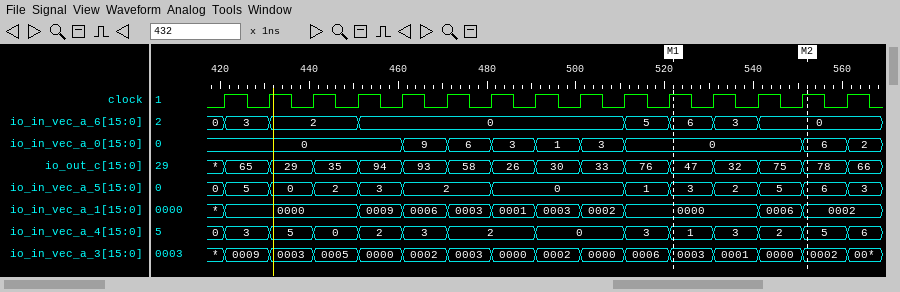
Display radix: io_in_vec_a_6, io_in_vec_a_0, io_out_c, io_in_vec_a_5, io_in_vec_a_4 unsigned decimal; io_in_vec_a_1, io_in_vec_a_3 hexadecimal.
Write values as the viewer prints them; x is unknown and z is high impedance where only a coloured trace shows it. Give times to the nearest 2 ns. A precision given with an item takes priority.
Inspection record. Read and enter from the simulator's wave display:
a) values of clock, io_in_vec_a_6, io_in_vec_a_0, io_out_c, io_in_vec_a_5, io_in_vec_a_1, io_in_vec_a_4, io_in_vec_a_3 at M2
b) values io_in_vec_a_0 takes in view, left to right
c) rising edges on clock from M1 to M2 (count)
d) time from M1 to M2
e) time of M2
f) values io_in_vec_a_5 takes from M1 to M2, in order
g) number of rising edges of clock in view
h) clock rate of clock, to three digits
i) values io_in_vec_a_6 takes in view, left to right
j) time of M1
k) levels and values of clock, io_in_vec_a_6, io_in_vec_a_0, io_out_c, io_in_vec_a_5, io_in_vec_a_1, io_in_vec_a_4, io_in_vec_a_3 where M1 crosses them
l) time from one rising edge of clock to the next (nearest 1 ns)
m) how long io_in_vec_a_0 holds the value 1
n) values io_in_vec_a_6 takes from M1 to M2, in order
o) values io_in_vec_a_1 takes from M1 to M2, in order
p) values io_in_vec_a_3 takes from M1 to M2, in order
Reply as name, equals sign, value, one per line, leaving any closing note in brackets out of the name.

values of clock, io_in_vec_a_6, io_in_vec_a_0, io_out_c, io_in_vec_a_5, io_in_vec_a_1, io_in_vec_a_4, io_in_vec_a_3 at M2 = clock=1, io_in_vec_a_6=0, io_in_vec_a_0=6, io_out_c=78, io_in_vec_a_5=6, io_in_vec_a_1=0002, io_in_vec_a_4=5, io_in_vec_a_3=0002
values io_in_vec_a_0 takes in view, left to right = 0, 9, 6, 3, 1, 3, 0, 6, 2
rising edges on clock from M1 to M2 = 3
time from M1 to M2 = 30 ns
time of M2 = 552 ns
values io_in_vec_a_5 takes from M1 to M2, in order = 3, 2, 5, 6
number of rising edges of clock in view = 15
clock rate of clock, to three digits = 100 MHz
values io_in_vec_a_6 takes in view, left to right = 0, 3, 2, 0, 5, 6, 3, 0
time of M1 = 522 ns
levels and values of clock, io_in_vec_a_6, io_in_vec_a_0, io_out_c, io_in_vec_a_5, io_in_vec_a_1, io_in_vec_a_4, io_in_vec_a_3 where M1 crosses them = clock=1, io_in_vec_a_6=6, io_in_vec_a_0=0, io_out_c=47, io_in_vec_a_5=3, io_in_vec_a_1=0000, io_in_vec_a_4=1, io_in_vec_a_3=0003
time from one rising edge of clock to the next = 10 ns
how long io_in_vec_a_0 holds the value 1 = 10 ns
values io_in_vec_a_6 takes from M1 to M2, in order = 6, 3, 0
values io_in_vec_a_1 takes from M1 to M2, in order = 0000, 0006, 0002
values io_in_vec_a_3 takes from M1 to M2, in order = 0003, 0001, 0000, 0002
